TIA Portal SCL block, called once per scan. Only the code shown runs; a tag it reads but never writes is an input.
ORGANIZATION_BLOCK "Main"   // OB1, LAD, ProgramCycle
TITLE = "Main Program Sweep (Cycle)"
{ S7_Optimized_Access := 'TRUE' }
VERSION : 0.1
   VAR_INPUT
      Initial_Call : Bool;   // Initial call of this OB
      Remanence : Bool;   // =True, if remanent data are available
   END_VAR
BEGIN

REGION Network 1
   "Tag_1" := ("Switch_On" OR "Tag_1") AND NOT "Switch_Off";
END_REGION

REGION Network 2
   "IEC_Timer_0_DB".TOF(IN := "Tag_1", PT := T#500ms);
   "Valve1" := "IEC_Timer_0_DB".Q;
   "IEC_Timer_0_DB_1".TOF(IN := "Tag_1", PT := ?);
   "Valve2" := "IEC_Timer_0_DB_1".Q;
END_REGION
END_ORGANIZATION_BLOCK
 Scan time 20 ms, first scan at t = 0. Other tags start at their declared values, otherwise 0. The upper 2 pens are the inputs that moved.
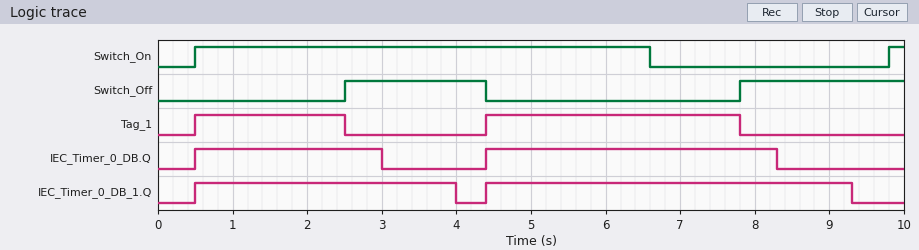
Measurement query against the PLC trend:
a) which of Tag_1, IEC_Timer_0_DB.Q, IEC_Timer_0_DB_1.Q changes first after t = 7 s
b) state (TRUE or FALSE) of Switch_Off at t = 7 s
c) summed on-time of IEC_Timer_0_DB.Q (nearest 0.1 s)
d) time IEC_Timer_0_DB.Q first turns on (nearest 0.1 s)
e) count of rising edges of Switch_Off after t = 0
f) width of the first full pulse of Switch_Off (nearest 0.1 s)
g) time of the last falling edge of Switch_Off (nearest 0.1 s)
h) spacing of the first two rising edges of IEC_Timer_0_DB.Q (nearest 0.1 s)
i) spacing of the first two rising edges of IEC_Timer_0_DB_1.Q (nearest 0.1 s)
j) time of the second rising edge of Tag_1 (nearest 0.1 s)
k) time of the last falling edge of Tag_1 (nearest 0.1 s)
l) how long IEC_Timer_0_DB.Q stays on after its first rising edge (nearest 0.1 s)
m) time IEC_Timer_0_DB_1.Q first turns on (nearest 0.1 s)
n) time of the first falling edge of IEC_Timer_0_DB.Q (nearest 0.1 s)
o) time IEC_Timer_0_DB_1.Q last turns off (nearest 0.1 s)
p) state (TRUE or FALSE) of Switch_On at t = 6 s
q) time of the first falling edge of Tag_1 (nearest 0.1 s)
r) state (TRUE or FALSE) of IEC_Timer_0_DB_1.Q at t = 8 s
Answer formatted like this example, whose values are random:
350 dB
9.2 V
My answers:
Tag_1
FALSE
6.4 s
0.5 s
2
1.9 s
4.4 s
3.9 s
3.9 s
4.4 s
7.8 s
2.5 s
0.5 s
3.0 s
9.3 s
TRUE
2.5 s
TRUE
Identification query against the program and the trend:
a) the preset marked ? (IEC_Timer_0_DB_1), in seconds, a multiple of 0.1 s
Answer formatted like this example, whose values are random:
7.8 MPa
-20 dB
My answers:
1.5 s
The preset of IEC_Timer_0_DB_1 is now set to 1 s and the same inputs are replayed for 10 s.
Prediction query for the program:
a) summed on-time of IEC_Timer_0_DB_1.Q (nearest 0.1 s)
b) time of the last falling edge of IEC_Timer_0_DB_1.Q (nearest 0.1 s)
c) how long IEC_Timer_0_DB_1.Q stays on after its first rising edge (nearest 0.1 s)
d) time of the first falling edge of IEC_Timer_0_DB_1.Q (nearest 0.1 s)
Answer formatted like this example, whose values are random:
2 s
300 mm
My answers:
7.4 s
8.8 s
3.0 s
3.5 s
